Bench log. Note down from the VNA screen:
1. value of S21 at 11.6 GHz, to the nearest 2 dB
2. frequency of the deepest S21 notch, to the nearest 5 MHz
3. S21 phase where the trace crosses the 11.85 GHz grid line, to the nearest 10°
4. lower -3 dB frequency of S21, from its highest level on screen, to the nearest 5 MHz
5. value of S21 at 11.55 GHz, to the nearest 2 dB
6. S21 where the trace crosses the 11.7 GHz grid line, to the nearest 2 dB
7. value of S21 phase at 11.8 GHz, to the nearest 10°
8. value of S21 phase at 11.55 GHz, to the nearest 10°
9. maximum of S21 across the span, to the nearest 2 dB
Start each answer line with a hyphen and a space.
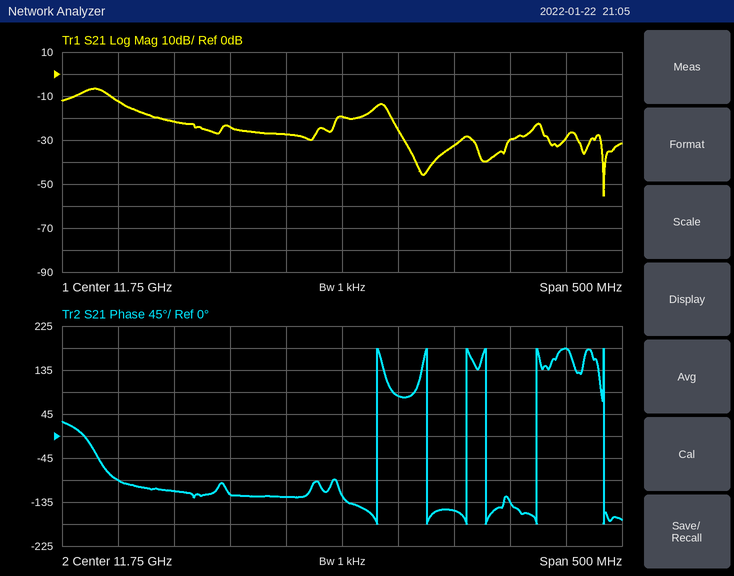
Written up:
- -22 dB
- 11.985 GHz
- -150°
- 11.515 GHz
- -12 dB
- -28 dB
- 80°
- -90°
- -6 dB
